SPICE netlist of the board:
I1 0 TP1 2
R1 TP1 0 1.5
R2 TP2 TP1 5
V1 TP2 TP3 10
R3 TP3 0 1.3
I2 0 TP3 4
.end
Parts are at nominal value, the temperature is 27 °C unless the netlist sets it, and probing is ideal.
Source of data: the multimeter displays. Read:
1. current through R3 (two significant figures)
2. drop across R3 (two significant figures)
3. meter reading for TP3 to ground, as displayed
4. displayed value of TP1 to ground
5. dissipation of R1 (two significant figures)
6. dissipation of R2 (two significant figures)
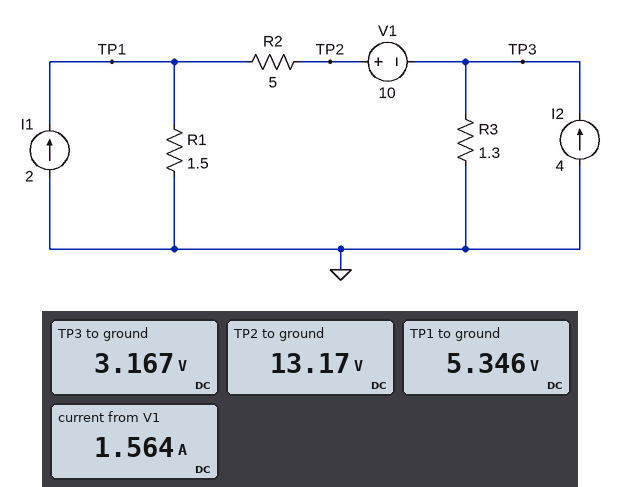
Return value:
2.4 A
3.2 V
3.167 V
5.346 V
19 W
12 W
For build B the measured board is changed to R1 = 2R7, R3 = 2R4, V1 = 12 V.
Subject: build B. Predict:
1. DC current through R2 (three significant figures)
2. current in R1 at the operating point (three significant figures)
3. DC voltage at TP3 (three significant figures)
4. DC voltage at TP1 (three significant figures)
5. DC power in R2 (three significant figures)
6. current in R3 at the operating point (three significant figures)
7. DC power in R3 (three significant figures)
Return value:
1.60 A
3.60 A
5.75 V
9.73 V
12.9 W
2.40 A
13.8 W
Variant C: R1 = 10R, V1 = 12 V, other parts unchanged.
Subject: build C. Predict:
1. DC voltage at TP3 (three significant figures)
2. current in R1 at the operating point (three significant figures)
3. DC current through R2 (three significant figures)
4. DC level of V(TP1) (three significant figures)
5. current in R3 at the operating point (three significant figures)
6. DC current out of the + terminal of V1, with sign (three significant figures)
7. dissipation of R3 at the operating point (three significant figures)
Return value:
5.42 V
1.83 A
172 mA
18.3 V
4.17 A
-172 mA
22.6 W
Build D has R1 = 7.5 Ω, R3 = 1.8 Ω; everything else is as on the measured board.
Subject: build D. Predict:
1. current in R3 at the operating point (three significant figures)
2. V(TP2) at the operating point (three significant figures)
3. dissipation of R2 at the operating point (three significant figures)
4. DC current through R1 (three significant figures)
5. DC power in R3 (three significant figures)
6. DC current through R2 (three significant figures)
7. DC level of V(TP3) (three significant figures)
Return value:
3.85 A
16.9 V
118 mW
2.15 A
26.6 W
154 mA
6.92 V
